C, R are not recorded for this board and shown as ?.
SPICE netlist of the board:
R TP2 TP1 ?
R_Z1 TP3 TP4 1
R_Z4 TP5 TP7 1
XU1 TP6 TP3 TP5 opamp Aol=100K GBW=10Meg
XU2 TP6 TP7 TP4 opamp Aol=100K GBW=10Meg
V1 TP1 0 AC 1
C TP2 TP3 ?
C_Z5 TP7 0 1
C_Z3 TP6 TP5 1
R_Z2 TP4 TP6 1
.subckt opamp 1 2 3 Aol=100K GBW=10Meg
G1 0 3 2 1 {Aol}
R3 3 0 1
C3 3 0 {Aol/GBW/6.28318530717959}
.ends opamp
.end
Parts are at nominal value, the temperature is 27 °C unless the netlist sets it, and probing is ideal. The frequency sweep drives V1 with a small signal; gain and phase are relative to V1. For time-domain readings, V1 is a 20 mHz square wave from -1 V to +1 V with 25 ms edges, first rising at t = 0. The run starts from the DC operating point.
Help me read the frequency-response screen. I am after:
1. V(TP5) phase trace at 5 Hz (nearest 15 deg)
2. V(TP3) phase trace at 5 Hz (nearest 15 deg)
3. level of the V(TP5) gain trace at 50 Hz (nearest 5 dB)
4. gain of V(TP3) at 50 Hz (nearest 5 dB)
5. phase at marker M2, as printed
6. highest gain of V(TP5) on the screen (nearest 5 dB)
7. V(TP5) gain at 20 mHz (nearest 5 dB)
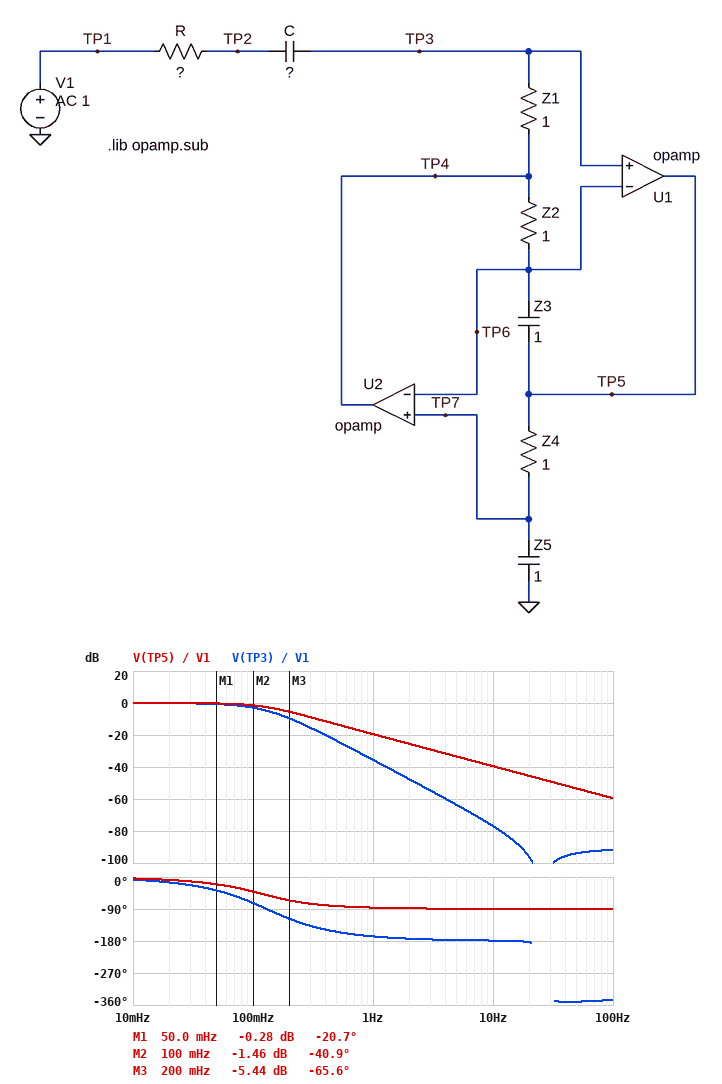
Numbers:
-90 deg
-180 deg
-55 dB
-95 dB
-40.9 deg
0 dB
0 dB
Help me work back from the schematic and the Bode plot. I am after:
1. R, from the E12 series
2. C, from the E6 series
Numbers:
1.5 Ω
470 mF
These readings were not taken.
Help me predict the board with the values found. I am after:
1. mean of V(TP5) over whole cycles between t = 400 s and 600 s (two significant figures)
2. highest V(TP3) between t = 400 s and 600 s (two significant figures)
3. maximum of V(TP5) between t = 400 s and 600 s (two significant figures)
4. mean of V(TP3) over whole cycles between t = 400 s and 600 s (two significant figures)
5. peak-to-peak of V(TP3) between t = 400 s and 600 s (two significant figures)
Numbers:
990 mV
2.0 V
2.0 V
990 mV
2.0 V
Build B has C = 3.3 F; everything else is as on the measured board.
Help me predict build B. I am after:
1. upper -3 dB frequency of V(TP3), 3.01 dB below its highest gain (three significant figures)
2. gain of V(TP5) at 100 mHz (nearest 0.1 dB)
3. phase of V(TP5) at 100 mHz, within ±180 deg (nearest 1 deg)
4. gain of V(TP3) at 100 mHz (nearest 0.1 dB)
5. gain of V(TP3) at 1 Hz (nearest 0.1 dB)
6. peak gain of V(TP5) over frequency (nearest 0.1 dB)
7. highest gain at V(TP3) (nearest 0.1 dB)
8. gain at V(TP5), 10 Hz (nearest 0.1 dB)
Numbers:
143 mHz
8.4 dB
7 deg
6.9 dB
-35.3 dB
14.4 dB
12.2 dB
-39.5 dB
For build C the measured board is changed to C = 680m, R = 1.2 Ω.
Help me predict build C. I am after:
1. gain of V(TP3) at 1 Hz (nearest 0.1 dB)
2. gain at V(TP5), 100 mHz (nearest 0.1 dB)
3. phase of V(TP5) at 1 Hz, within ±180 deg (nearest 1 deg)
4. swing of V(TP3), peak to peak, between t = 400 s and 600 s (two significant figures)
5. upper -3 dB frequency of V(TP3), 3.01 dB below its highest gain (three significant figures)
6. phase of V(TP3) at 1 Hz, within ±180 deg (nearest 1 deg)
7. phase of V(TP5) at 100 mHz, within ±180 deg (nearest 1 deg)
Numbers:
-33.5 dB
0.9 dB
-88 deg
2.2 V
152 mHz
-169 deg
-28 deg
